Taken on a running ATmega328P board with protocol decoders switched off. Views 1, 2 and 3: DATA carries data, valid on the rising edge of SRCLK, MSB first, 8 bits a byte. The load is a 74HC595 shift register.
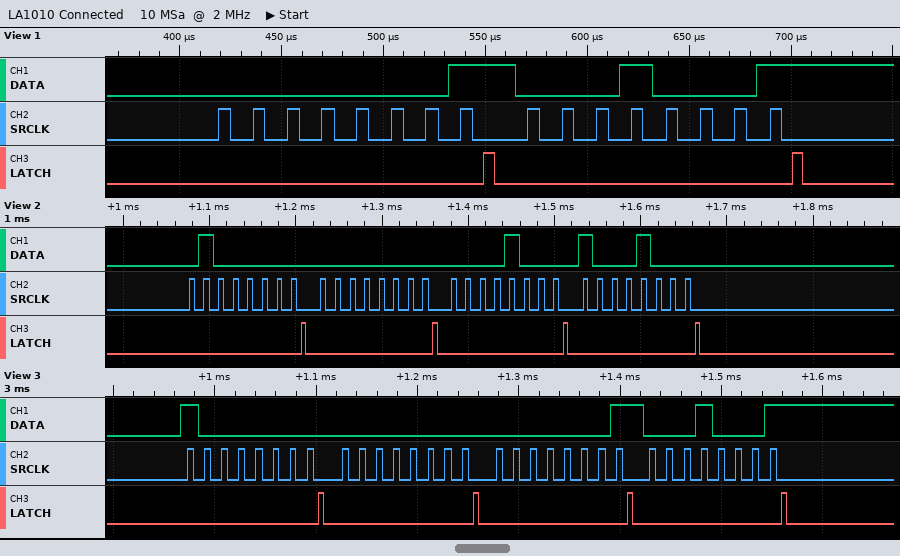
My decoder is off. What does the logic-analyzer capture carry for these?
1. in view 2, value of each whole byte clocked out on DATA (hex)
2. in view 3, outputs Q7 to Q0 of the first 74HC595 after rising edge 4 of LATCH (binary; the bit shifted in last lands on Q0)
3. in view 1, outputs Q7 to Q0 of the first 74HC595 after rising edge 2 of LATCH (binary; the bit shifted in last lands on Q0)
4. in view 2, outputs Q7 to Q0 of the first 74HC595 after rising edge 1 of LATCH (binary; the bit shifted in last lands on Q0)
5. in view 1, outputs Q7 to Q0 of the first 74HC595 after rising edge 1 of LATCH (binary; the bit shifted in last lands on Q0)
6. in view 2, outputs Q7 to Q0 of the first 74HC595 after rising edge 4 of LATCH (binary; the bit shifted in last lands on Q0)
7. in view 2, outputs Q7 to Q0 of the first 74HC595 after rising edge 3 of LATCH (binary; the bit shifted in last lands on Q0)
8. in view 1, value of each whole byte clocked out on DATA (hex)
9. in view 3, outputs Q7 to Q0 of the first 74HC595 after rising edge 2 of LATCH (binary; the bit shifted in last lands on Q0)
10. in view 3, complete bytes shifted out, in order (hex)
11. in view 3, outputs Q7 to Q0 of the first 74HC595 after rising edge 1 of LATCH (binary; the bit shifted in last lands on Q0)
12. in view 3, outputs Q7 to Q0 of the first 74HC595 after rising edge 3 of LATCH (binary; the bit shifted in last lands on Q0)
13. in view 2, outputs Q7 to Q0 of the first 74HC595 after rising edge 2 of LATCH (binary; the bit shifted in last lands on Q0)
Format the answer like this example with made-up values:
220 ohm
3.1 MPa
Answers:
40 00 08 88
00010001
00010001
01000000
00000001
10001000
00001000
01 11
00000000
0x80 0x00 0x01 0x11
10000000
00000001
00000000
